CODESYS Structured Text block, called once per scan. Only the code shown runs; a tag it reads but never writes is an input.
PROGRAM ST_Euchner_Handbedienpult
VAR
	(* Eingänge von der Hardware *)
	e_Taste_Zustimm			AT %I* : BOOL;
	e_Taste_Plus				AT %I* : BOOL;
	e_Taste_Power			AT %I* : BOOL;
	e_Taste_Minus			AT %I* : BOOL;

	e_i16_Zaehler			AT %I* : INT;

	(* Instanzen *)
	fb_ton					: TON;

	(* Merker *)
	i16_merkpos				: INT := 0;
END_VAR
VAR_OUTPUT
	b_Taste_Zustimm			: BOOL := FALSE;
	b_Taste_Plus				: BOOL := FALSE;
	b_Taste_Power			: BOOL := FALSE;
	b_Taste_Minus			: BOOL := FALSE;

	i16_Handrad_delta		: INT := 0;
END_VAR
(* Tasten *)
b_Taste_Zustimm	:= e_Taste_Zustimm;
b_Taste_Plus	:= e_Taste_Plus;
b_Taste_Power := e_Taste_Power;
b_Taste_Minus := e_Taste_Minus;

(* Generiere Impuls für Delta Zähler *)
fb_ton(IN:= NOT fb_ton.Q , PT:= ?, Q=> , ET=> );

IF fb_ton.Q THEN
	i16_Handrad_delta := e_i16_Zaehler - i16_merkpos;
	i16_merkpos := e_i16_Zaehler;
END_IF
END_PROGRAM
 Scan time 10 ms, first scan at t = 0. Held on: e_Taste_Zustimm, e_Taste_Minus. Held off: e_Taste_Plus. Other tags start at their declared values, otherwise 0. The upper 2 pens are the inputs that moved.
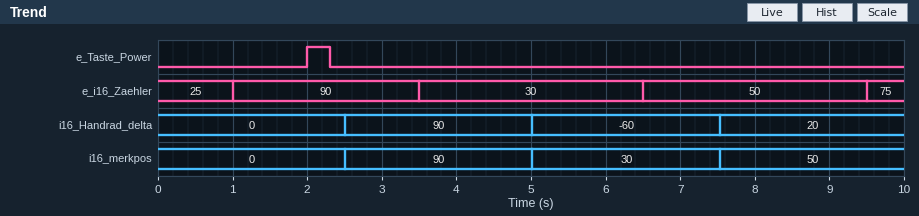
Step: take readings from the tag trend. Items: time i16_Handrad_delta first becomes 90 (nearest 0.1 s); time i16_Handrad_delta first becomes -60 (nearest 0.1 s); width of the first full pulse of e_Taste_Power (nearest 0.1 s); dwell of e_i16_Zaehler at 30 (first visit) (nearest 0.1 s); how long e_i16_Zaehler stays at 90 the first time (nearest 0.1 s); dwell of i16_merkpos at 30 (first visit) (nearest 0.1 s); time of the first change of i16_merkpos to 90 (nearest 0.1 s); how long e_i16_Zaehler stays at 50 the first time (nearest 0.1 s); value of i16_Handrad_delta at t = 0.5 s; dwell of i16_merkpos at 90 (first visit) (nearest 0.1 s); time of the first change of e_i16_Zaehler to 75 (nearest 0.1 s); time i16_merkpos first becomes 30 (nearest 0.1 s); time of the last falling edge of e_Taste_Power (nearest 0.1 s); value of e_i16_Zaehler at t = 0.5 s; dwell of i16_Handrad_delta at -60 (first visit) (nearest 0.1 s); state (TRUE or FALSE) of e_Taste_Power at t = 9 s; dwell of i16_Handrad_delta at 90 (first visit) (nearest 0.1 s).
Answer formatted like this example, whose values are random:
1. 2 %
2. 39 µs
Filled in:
1. 2.5 s
2. 5.0 s
3. 0.3 s
4. 3.0 s
5. 2.5 s
6. 2.5 s
7. 2.5 s
8. 3.0 s
9. 0
10. 2.5 s
11. 9.5 s
12. 5.0 s
13. 2.3 s
14. 25
15. 2.5 s
16. FALSE
17. 2.5 s
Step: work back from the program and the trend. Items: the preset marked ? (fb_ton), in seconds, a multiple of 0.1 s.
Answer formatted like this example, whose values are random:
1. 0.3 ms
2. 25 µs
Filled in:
1. 2.5 s
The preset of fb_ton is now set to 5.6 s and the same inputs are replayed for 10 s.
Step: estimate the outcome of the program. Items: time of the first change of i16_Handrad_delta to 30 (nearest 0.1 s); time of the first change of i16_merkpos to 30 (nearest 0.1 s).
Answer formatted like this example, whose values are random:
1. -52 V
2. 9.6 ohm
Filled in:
1. 5.6 s
2. 5.6 s
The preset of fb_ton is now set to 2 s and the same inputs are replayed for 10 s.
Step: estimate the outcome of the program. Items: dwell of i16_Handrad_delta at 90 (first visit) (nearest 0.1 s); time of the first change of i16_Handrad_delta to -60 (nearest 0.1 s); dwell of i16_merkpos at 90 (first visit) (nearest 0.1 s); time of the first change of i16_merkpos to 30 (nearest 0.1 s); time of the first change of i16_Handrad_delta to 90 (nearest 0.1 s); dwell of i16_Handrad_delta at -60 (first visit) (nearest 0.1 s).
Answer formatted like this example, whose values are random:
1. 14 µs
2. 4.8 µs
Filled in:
1. 2.0 s
2. 4.0 s
3. 2.0 s
4. 4.0 s
5. 2.0 s
6. 2.0 s
